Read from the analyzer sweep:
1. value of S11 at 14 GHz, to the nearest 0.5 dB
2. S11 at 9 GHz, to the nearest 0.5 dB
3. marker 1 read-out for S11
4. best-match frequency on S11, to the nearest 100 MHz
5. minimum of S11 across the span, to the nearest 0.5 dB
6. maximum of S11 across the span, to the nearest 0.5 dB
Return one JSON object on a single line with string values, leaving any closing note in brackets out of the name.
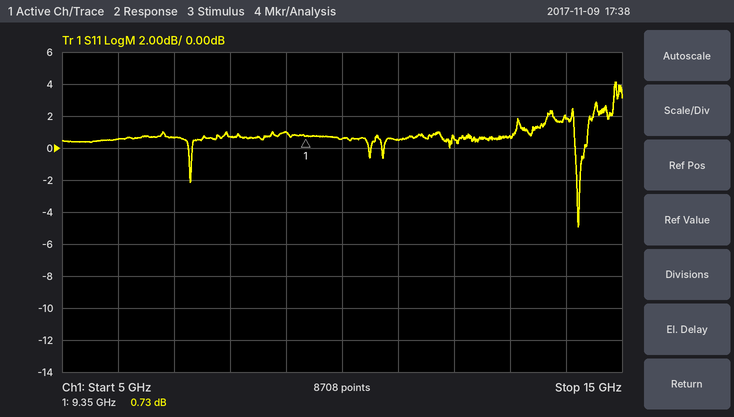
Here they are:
{"value of S11 at 14 GHz, to the nearest 0.5 dB": "2.0 dB", "S11 at 9 GHz, to the nearest 0.5 dB": "1.0 dB", "marker 1 read-out for S11": "0.73 dB", "best-match frequency on S11, to the nearest 100 MHz": "14.2 GHz", "minimum of S11 across the span, to the nearest 0.5 dB": "-5.0 dB", "maximum of S11 across the span, to the nearest 0.5 dB": "4.0 dB"}
